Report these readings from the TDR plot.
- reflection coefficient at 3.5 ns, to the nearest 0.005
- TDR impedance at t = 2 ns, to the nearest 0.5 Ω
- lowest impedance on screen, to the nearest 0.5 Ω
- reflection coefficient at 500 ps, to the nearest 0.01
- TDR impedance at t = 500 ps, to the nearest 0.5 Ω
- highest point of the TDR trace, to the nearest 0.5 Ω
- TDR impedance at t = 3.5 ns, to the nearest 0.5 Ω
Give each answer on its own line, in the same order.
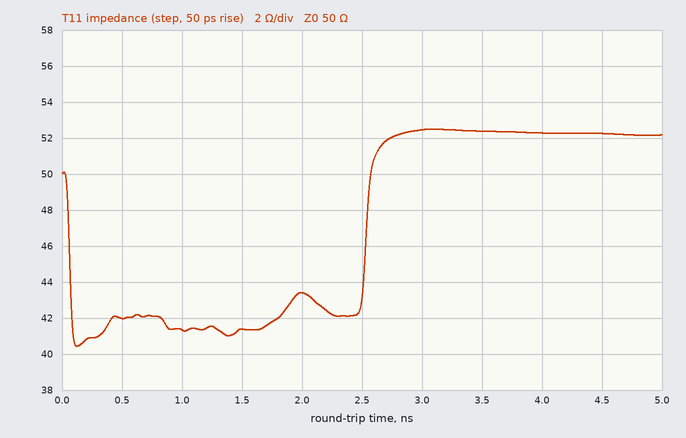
+0.025
43.5 Ω
40.5 Ω
-0.09
42.0 Ω
52.5 Ω
52.5 Ω
